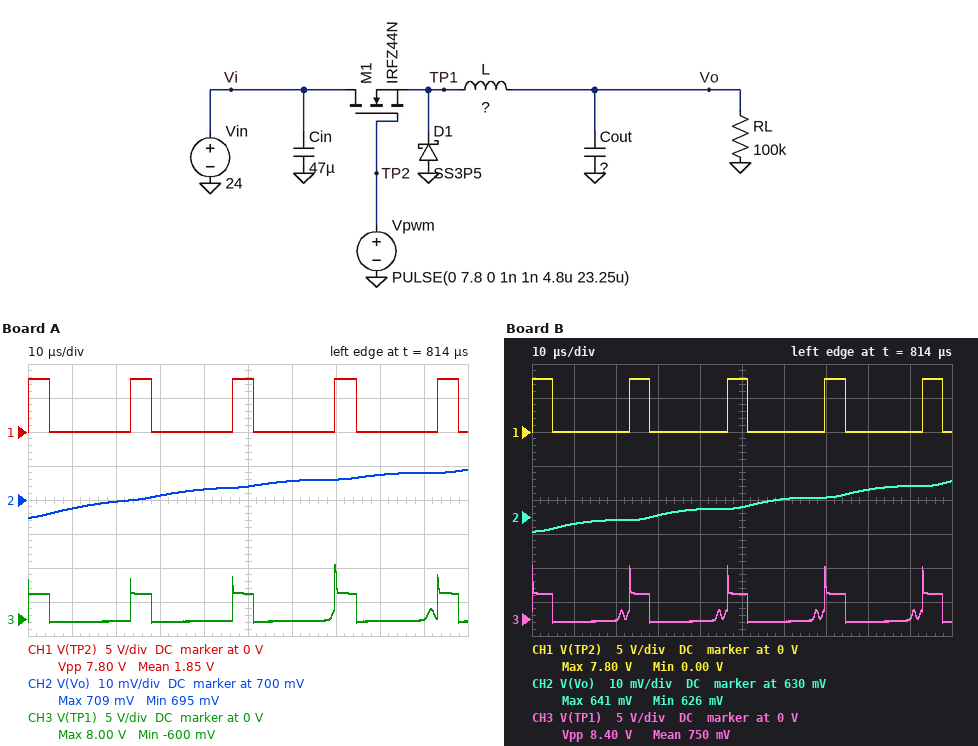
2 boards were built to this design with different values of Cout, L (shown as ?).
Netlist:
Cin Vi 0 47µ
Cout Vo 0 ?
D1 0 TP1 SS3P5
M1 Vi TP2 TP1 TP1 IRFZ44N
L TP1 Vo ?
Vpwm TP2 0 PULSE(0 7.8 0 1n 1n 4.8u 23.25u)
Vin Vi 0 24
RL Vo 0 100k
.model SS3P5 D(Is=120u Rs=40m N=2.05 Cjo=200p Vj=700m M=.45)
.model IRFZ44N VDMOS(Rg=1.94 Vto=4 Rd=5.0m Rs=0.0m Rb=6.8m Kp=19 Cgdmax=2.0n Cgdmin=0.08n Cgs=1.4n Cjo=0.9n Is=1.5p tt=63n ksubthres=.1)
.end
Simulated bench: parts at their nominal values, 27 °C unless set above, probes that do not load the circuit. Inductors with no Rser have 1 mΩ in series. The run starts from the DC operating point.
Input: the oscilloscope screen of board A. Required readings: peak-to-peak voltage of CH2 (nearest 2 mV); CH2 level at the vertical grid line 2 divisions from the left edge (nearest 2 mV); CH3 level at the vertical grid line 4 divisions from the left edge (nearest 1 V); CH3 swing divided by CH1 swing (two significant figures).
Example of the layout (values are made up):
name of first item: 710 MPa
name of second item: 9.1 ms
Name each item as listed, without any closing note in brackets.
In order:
peak-to-peak voltage of CH2: 14 mV
CH2 level at the vertical grid line 2 divisions from the left edge: 700 mV
CH3 level at the vertical grid line 4 divisions from the left edge: 0 V
CH3 swing divided by CH1 swing: 1.1
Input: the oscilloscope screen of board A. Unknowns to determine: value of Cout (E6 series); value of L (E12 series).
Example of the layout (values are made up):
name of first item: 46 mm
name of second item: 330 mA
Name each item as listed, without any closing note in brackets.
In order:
value of Cout: 680 µF
value of L: 120 µH
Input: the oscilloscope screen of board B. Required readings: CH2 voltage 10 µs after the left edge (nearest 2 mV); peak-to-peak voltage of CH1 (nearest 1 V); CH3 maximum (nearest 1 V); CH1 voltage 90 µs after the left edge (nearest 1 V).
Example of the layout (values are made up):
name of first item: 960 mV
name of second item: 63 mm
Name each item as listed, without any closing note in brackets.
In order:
CH2 voltage 10 µs after the left edge: 628 mV
peak-to-peak voltage of CH1: 8 V
CH3 maximum: 8 V
CH1 voltage 90 µs after the left edge: 0 V
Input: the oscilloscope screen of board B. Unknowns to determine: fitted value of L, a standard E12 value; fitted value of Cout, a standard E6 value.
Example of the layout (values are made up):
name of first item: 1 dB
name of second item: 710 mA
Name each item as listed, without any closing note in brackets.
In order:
fitted value of L, a standard E12 value: 47 µH
fitted value of Cout, a standard E6 value: 1 mF
